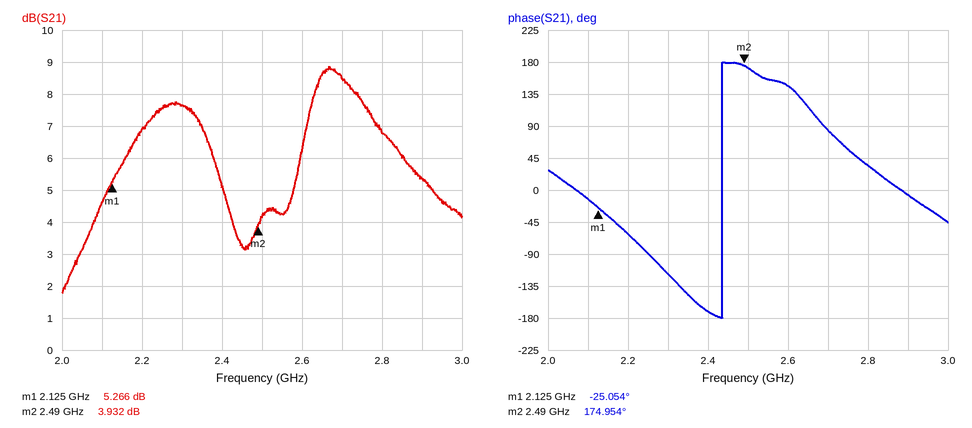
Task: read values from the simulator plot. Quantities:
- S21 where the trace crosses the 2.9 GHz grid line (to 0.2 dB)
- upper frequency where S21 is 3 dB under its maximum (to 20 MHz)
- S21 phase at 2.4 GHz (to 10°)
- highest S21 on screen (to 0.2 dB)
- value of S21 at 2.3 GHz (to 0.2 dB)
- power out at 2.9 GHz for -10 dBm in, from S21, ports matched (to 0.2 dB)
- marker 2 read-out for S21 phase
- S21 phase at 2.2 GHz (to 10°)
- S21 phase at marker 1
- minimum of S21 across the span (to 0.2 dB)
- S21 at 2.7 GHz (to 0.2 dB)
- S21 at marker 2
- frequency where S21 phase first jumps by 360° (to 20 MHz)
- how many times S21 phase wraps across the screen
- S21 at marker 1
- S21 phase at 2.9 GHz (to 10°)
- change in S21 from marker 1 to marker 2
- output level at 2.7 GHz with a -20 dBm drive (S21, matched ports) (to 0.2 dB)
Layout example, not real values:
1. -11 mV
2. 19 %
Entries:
1. 5.4 dB
2. 2.86 GHz
3. -170°
4. 8.8 dB
5. 7.6 dB
6. -4.6 dBm
7. 174.954°
8. -60°
9. -25.054°
10. 1.8 dB
11. 8.4 dB
12. 3.932 dB
13. 2.44 GHz
14. 1
15. 5.266 dB
16. -10°
17. -1.334 dB
18. -11.6 dBm
